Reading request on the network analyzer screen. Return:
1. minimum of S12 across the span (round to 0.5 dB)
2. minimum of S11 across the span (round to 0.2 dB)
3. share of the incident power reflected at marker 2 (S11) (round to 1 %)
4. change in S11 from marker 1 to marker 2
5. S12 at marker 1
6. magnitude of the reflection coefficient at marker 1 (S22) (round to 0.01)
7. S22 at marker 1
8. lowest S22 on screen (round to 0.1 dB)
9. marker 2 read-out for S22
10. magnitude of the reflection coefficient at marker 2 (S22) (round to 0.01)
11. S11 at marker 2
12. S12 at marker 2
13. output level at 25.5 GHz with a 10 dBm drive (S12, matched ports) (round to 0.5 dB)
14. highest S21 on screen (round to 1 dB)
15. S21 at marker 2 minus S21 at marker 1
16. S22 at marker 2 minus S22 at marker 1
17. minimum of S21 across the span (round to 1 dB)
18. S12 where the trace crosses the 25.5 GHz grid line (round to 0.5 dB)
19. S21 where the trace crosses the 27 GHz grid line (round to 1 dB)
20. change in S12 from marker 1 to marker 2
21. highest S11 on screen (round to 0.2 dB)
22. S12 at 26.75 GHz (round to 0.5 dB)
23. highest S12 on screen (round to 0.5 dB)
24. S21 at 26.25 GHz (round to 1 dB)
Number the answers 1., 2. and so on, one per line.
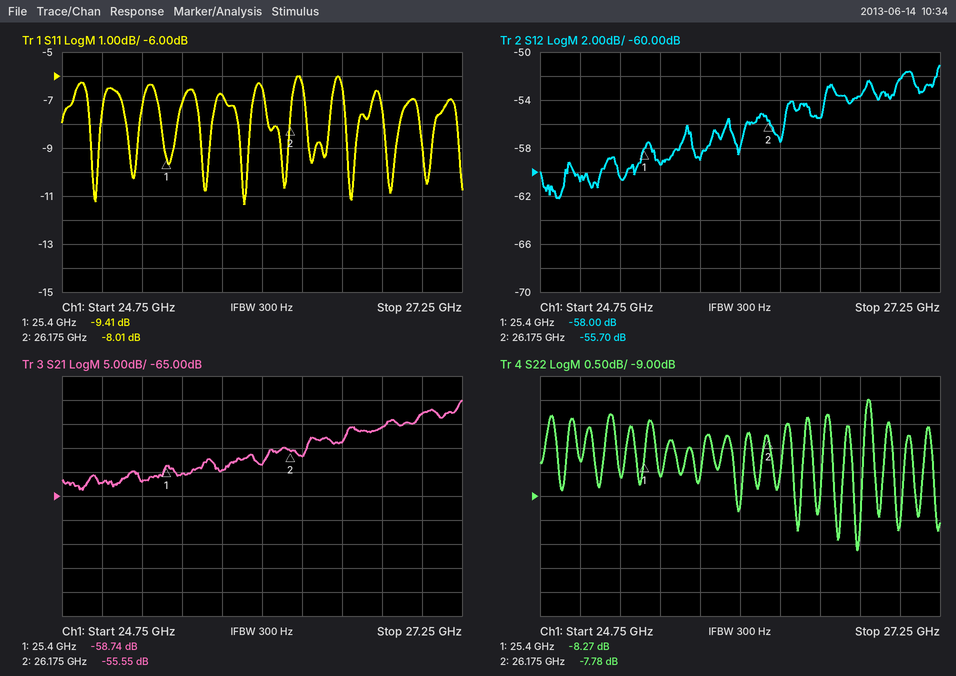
1. -62.0 dB
2. -11.4 dB
3. 16 %
4. 1.40 dB
5. -58.00 dB
6. 0.39
7. -8.27 dB
8. -10.1 dB
9. -7.78 dB
10. 0.41
11. -8.01 dB
12. -55.70 dB
13. -49.5 dBm
14. -45 dB
15. 3.19 dB
16. 0.49 dB
17. -64 dB
18. -59.5 dB
19. -48 dB
20. 2.30 dB
21. -6.0 dB
22. -53.5 dB
23. -51.0 dB
24. -57 dB
